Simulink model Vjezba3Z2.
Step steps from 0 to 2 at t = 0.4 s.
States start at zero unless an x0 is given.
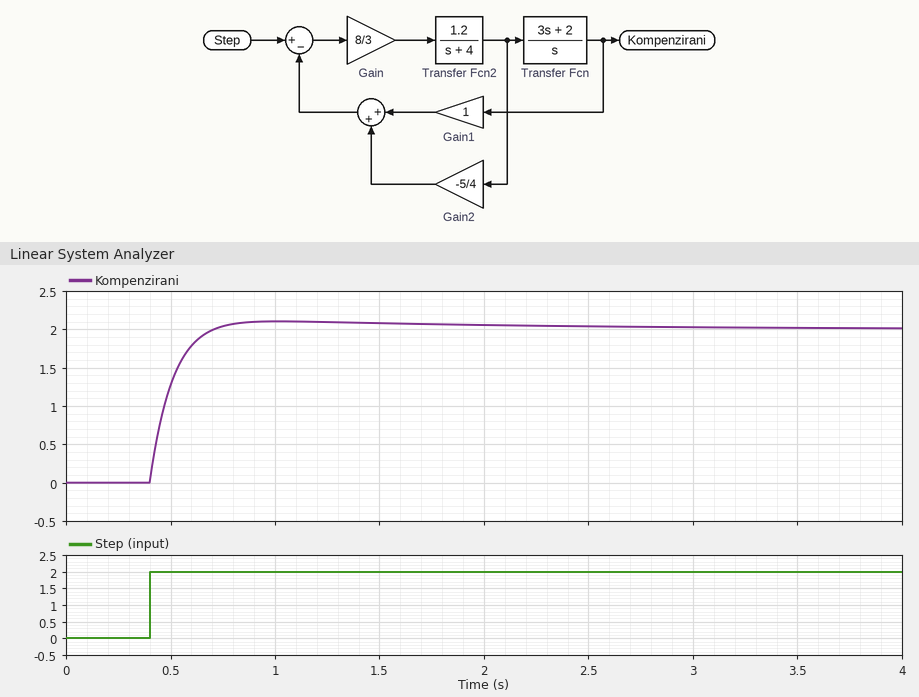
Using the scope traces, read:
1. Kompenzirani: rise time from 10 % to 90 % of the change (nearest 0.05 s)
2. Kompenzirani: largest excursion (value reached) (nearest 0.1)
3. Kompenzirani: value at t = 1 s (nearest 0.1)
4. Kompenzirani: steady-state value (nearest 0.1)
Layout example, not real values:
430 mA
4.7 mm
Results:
0.20 s
2.1
2.1
2.0
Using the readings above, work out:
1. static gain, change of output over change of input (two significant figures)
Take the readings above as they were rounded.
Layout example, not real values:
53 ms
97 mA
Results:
1.0
